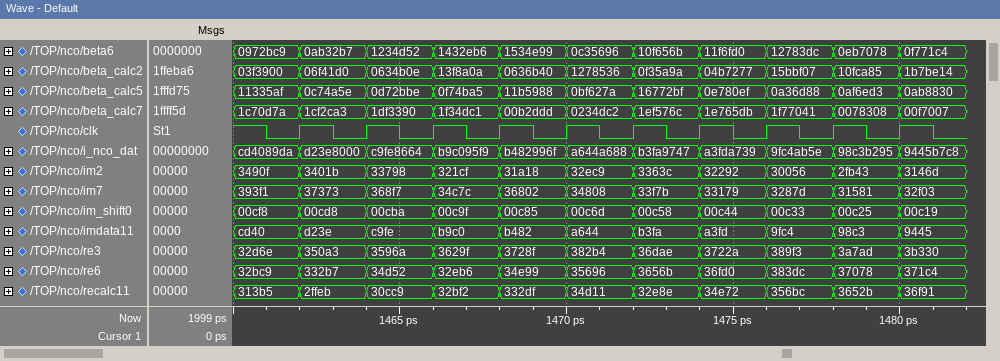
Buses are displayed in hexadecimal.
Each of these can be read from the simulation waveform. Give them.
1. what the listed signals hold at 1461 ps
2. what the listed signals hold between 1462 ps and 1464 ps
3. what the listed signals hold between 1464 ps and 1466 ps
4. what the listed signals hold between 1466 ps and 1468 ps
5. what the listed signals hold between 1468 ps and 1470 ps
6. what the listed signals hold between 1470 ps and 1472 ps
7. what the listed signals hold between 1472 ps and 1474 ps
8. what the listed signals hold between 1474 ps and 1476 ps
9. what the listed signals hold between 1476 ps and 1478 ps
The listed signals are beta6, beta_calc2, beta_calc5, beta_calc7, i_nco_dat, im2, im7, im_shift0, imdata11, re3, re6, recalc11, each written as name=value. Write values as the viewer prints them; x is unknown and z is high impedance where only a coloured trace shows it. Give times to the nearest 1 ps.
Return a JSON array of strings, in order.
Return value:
["beta6=0972bc9, beta_calc2=03f3900, beta_calc5=11335af, beta_calc7=1c70d7a, i_nco_dat=cd4089da, im2=3490f, im7=393f1, im_shift0=00cf8, imdata11=cd40, re3=32d6e, re6=32bc9, recalc11=313b5", "beta6=0ab32b7, beta_calc2=06f41d0, beta_calc5=0c74a5e, beta_calc7=1cf2ca3, i_nco_dat=d23e8000, im2=3401b, im7=37373, im_shift0=00cd8, imdata11=d23e, re3=350a3, re6=332b7, recalc11=2ffeb", "beta6=1234d52, beta_calc2=0634b0e, beta_calc5=0d72bbe, beta_calc7=1df3390, i_nco_dat=c9fe8664, im2=33798, im7=368f7, im_shift0=00cba, imdata11=c9fe, re3=3596a, re6=34d52, recalc11=30cc9", "beta6=1432eb6, beta_calc2=13f8a0a, beta_calc5=0f74ba5, beta_calc7=1f34dc1, i_nco_dat=b9c095f9, im2=321cf, im7=34c7c, im_shift0=00c9f, imdata11=b9c0, re3=3629f, re6=32eb6, recalc11=32bf2", "beta6=1534e99, beta_calc2=0636b40, beta_calc5=11b5988, beta_calc7=00b2ddd, i_nco_dat=b482996f, im2=31a18, im7=36802, im_shift0=00c85, imdata11=b482, re3=3728f, re6=34e99, recalc11=332df", "beta6=0c35696, beta_calc2=1278536, beta_calc5=0bf627a, beta_calc7=0234dc2, i_nco_dat=a644a688, im2=32ec9, im7=34808, im_shift0=00c6d, imdata11=a644, re3=382b4, re6=35696, recalc11=34d11", "beta6=10f656b, beta_calc2=0f35a9a, beta_calc5=16772bf, beta_calc7=1ef576c, i_nco_dat=b3fa9747, im2=3363c, im7=33f7b, im_shift0=00c58, imdata11=b3fa, re3=36dae, re6=3656b, recalc11=32e8e", "beta6=11f6fd0, beta_calc2=04b7277, beta_calc5=0e780ef, beta_calc7=1e765db, i_nco_dat=a3fda739, im2=32292, im7=33179, im_shift0=00c44, imdata11=a3fd, re3=3722a, re6=36fd0, recalc11=34e72", "beta6=12783dc, beta_calc2=15bbf07, beta_calc5=0a36d88, beta_calc7=1f77041, i_nco_dat=9fc4ab5e, im2=30056, im7=3287d, im_shift0=00c33, imdata11=9fc4, re3=389f3, re6=383dc, recalc11=356bc"]
